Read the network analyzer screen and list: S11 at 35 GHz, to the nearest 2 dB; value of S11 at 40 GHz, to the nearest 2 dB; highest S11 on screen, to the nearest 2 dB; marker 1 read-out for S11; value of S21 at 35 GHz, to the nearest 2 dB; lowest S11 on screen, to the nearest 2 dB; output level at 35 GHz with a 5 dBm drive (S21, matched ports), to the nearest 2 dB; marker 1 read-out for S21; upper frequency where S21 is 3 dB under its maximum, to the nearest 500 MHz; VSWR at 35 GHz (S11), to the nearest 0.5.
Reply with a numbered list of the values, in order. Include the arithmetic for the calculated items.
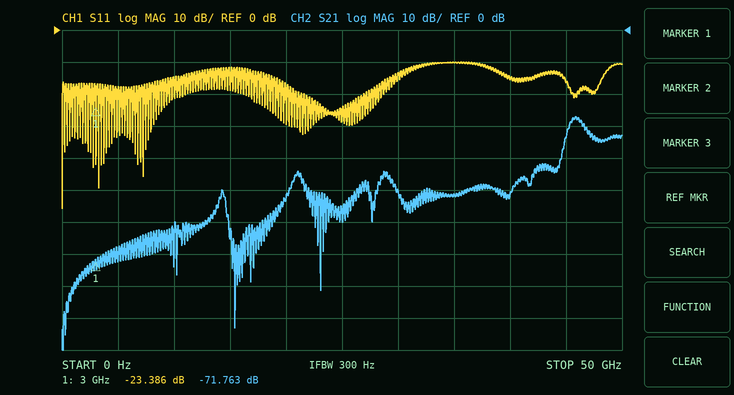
1. -10 dB
2. -16 dB
3. -10 dB
4. -23.386 dB
5. -52 dB
6. -56 dB
7. 5 dBm + (-52 dB) = -46 dBm
8. -71.763 dB
9. 46.5 GHz
10. |Γ| = 10^(-10/20) = 0.3162; VSWR = (1 + 0.3162)/(1 − 0.3162) ≈ 1.92, so 2.0 to the nearest 0.5
